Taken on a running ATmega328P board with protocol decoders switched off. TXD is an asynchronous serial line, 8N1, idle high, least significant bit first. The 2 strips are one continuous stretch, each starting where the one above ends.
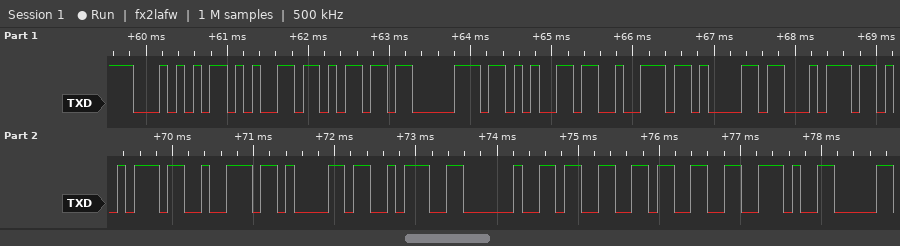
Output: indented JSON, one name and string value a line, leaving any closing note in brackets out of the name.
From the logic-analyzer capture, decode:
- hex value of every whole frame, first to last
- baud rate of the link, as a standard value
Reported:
{
  "hex value of every whole frame, first to last": "0x54 0x65 0x6D 0x70 0x65 0x72 0x61 0x74 0x75 0x72 0x61 0x3A 0x20 0x33 0x33 0x2E",
  "baud rate of the link, as a standard value": "9600 baud"
}
